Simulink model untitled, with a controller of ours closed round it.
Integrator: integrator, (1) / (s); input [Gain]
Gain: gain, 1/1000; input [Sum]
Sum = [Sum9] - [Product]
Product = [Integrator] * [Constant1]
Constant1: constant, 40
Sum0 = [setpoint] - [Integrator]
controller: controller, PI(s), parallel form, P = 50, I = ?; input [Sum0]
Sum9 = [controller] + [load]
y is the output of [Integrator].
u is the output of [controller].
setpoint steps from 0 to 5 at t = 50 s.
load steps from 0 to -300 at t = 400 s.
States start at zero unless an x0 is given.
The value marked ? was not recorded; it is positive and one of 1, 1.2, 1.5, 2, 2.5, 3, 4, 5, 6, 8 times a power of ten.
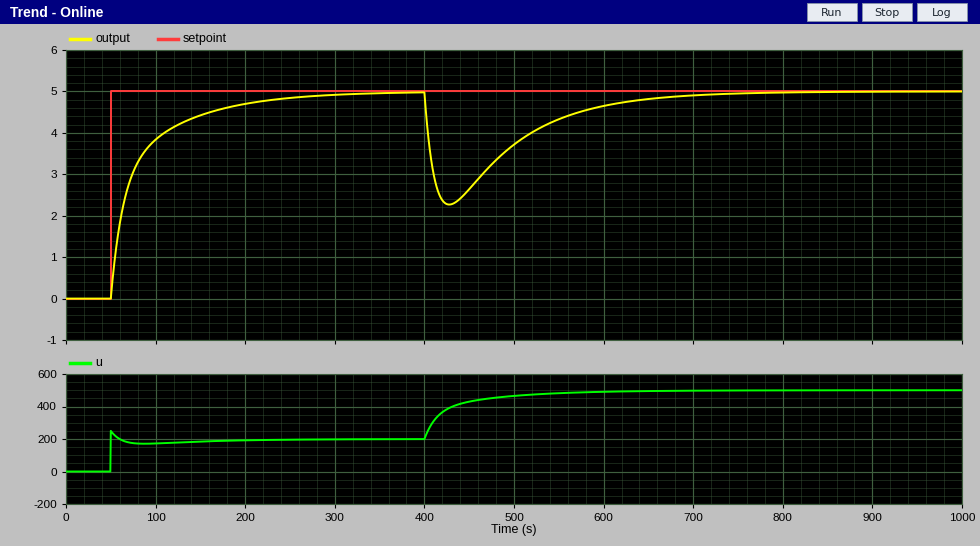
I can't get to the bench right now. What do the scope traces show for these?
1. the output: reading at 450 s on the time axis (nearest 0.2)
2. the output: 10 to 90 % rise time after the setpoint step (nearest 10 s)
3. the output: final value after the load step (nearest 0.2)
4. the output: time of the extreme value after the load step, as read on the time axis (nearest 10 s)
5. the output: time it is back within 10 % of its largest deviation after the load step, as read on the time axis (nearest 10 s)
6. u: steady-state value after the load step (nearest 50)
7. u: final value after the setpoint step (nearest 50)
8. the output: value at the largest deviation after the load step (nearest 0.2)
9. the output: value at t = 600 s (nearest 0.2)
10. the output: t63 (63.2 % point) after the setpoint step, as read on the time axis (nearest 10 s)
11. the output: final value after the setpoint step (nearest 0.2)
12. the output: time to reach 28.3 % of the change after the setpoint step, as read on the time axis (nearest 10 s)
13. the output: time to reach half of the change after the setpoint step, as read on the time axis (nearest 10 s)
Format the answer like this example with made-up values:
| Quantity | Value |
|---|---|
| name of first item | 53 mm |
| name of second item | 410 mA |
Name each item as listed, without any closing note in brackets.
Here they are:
| Quantity | Value |
|---|---|
| the output: reading at 450 s on the time axis | 2.6 |
| the output: 10 to 90 % rise time after the setpoint step | 110 s |
| the output: final value after the load step | 5.0 |
| the output: time of the extreme value after the load step, as read on the time axis | 430 s |
| the output: time it is back within 10 % of its largest deviation after the load step, as read on the time axis | 620 s |
| u: steady-state value after the load step | 500 |
| u: final value after the setpoint step | 200 |
| the output: value at the largest deviation after the load step | 2.2 |
| the output: value at t = 600 s | 4.6 |
| the output: t63 (63.2 % point) after the setpoint step, as read on the time axis | 80 s |
| the output: final value after the setpoint step | 5.0 |
| the output: time to reach 28.3 % of the change after the setpoint step, as read on the time axis | 60 s |
| the output: time to reach half of the change after the setpoint step, as read on the time axis | 70 s |
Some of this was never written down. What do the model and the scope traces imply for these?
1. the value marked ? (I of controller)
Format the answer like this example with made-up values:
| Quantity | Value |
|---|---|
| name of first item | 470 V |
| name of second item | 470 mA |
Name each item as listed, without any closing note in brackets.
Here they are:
| Quantity | Value |
|---|---|
| the value marked ? | 1 |
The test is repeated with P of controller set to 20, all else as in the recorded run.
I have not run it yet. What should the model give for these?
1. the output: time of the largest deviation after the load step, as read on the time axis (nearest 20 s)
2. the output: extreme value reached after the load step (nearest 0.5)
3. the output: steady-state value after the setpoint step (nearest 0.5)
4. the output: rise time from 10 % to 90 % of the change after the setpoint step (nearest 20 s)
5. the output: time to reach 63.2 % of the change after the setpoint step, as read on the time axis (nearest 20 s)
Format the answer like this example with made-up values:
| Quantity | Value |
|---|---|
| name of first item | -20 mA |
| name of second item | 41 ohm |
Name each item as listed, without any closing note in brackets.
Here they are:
| Quantity | Value |
|---|---|
| the output: time of the largest deviation after the load step, as read on the time axis | 440 s |
| the output: extreme value reached after the load step | 1.5 |
| the output: steady-state value after the setpoint step | 5.0 |
| the output: rise time from 10 % to 90 % of the change after the setpoint step | 80 s |
| the output: time to reach 63.2 % of the change after the setpoint step, as read on the time axis | 100 s |
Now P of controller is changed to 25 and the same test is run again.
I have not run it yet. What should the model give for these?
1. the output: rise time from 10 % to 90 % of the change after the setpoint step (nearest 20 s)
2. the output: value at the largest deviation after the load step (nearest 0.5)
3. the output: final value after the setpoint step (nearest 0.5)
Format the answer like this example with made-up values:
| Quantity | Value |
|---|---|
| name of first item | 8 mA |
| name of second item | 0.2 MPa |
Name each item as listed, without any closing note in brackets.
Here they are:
| Quantity | Value |
|---|---|
| the output: rise time from 10 % to 90 % of the change after the setpoint step | 80 s |
| the output: value at the largest deviation after the load step | 1.5 |
| the output: final value after the setpoint step | 5.0 |
